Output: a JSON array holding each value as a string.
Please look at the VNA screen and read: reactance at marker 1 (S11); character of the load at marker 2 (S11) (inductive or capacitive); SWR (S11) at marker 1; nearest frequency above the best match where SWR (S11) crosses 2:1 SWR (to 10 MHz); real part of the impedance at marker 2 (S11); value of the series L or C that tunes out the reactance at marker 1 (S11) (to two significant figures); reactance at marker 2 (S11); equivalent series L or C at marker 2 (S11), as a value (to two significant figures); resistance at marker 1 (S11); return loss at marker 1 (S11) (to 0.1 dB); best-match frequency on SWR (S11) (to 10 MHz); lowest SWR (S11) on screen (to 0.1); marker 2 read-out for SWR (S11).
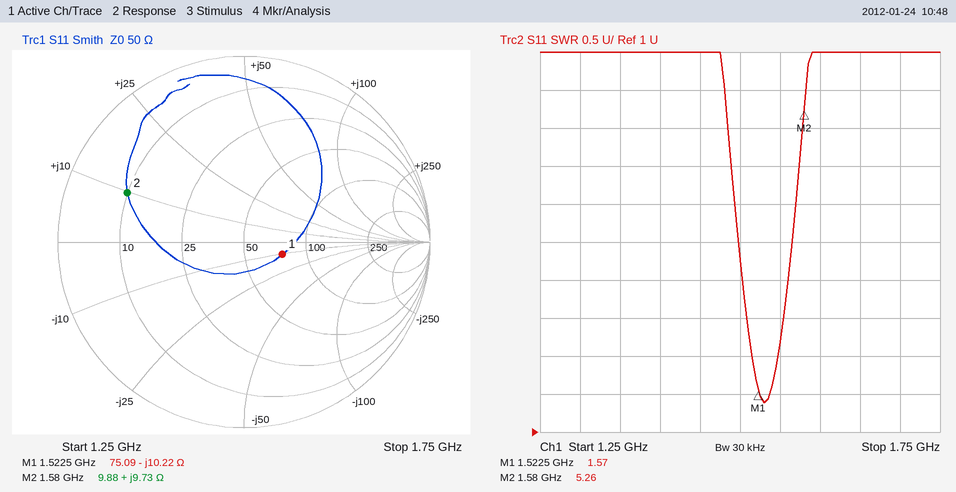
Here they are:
["-10.22 Ω", "inductive", "1.57", "1.55 GHz", "9.88 Ω", "1.1 nH", "+9.73 Ω", "980 pH", "75.09 Ω", "13.3 dB", "1.53 GHz", "1.4", "5.26"]
